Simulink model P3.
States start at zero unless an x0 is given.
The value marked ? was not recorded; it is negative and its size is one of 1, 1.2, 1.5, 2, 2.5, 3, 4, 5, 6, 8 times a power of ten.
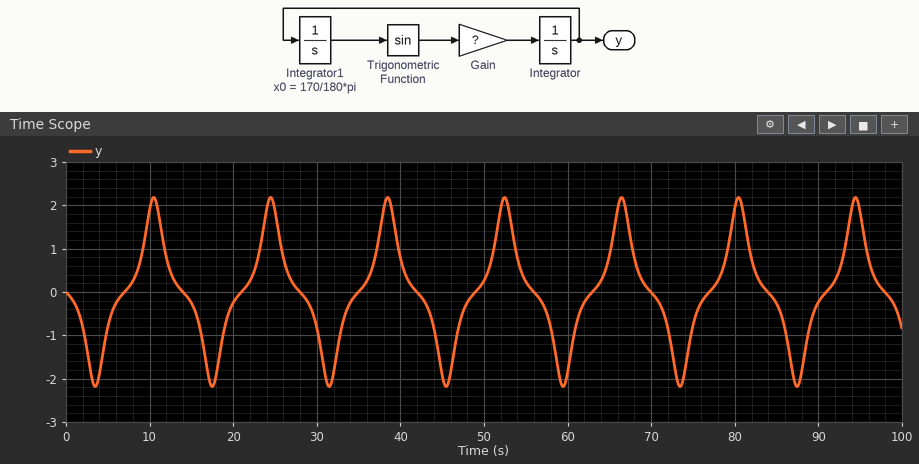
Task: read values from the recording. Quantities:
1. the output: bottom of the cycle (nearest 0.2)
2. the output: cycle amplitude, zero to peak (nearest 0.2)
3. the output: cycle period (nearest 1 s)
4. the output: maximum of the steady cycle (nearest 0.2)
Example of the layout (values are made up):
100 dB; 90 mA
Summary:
-2.2; 2.2; 14 s; 2.2
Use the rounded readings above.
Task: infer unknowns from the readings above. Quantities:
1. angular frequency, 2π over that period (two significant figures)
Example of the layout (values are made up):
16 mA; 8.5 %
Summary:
0.45 rad/s
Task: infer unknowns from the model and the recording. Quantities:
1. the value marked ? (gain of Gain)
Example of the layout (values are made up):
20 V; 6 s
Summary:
-1.2
